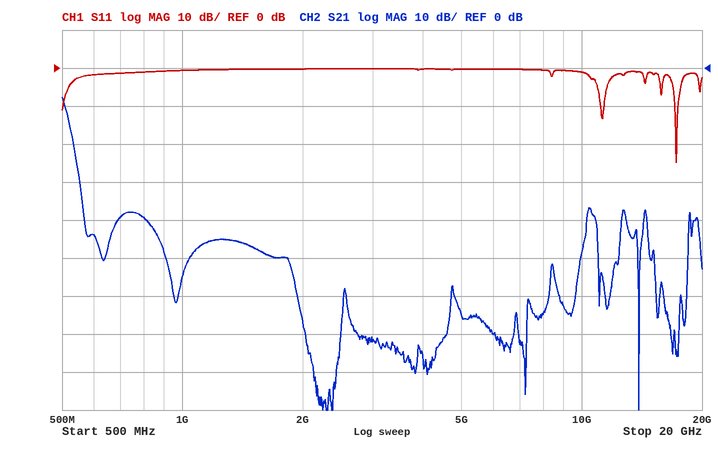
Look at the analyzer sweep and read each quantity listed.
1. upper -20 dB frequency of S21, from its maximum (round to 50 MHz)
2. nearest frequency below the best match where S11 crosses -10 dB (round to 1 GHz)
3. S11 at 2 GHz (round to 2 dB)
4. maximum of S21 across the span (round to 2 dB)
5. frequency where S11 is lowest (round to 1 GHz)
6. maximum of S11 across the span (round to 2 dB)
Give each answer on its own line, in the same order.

550 MHz
17 GHz
0 dB
-8 dB
17 GHz
0 dB
